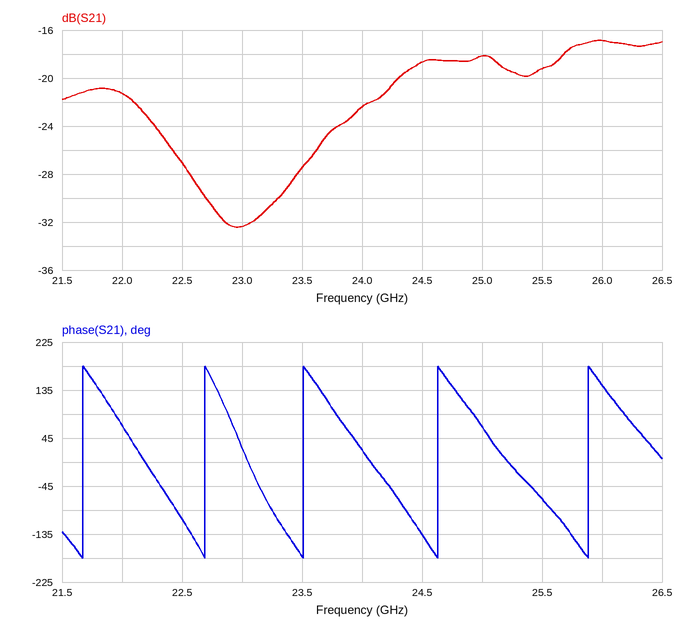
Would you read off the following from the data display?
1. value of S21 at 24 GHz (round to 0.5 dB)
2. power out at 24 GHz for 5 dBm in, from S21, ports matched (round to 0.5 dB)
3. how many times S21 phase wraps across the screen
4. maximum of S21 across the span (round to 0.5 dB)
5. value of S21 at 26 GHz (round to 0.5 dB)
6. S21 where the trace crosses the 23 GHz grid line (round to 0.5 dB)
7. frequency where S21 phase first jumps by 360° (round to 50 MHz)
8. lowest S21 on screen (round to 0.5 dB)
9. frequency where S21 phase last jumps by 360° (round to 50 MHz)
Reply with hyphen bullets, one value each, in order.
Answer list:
- -22.5 dB
- -17.5 dBm
- 5
- -17.0 dB
- -17.0 dB
- -32.5 dB
- 21.65 GHz
- -32.5 dB
- 25.90 GHz
